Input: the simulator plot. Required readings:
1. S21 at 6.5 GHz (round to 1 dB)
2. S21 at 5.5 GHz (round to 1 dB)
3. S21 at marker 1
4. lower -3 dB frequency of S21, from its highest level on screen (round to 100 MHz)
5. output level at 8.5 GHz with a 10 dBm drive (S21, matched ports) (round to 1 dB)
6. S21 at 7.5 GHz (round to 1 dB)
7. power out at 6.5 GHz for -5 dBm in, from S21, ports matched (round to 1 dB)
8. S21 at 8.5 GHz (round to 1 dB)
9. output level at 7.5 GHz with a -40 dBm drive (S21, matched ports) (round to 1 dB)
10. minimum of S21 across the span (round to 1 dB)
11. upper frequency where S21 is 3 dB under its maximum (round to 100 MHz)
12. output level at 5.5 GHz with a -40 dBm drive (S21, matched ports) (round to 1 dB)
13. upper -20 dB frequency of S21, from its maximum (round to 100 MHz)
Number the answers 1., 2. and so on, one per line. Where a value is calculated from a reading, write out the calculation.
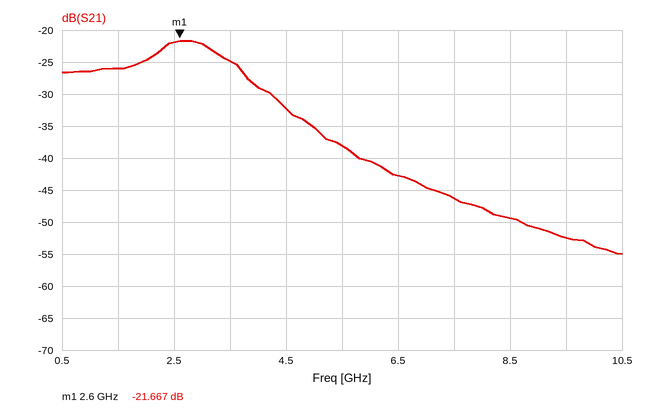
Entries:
1. -43 dB
2. -38 dB
3. -21.667 dB
4. 2.0 GHz
5. 10 dBm + (-49 dB) = -39 dBm
6. -46 dB
7. -5 dBm + (-43 dB) = -48 dBm
8. -49 dB
9. -40 dBm + (-46 dB) = -86 dBm
10. -55 dB
11. 3.5 GHz
12. -40 dBm + (-38 dB) = -78 dBm
13. 6.3 GHz
